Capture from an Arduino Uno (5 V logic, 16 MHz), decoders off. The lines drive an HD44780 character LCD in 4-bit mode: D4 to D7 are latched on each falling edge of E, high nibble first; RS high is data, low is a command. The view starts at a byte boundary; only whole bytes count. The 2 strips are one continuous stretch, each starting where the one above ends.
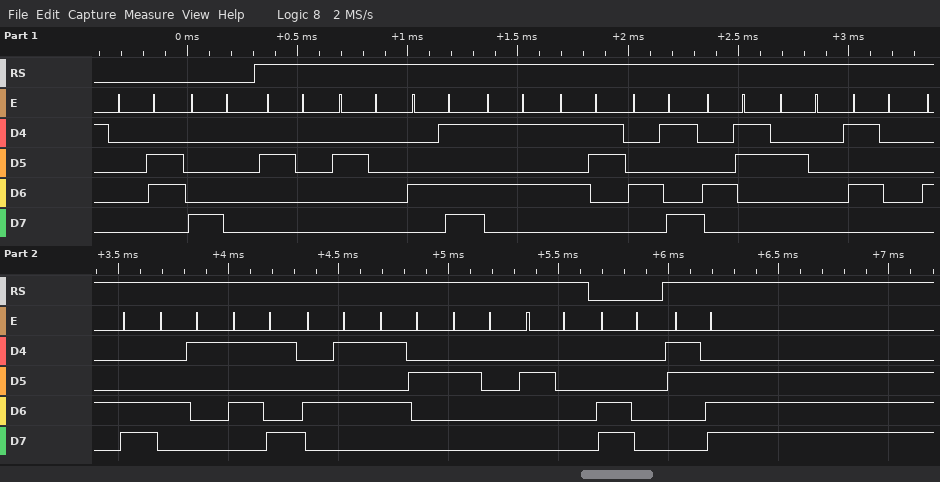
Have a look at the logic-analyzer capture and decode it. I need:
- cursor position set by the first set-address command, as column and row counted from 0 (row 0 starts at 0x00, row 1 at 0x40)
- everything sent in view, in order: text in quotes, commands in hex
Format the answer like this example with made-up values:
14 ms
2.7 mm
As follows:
column 0, row 0
0x06 0x80 "  MUSIC PLAYER  " 0xC0 ">"
